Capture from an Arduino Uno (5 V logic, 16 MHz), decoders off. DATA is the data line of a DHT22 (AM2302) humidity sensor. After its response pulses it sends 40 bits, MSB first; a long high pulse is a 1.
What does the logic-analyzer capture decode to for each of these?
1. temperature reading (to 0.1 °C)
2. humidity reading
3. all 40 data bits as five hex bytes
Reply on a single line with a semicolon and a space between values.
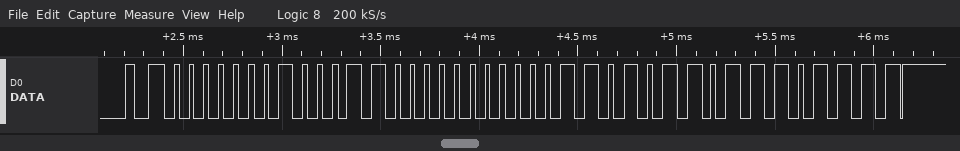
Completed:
21.4 °C; 28.0 %; 01 18 00 D6 EF
